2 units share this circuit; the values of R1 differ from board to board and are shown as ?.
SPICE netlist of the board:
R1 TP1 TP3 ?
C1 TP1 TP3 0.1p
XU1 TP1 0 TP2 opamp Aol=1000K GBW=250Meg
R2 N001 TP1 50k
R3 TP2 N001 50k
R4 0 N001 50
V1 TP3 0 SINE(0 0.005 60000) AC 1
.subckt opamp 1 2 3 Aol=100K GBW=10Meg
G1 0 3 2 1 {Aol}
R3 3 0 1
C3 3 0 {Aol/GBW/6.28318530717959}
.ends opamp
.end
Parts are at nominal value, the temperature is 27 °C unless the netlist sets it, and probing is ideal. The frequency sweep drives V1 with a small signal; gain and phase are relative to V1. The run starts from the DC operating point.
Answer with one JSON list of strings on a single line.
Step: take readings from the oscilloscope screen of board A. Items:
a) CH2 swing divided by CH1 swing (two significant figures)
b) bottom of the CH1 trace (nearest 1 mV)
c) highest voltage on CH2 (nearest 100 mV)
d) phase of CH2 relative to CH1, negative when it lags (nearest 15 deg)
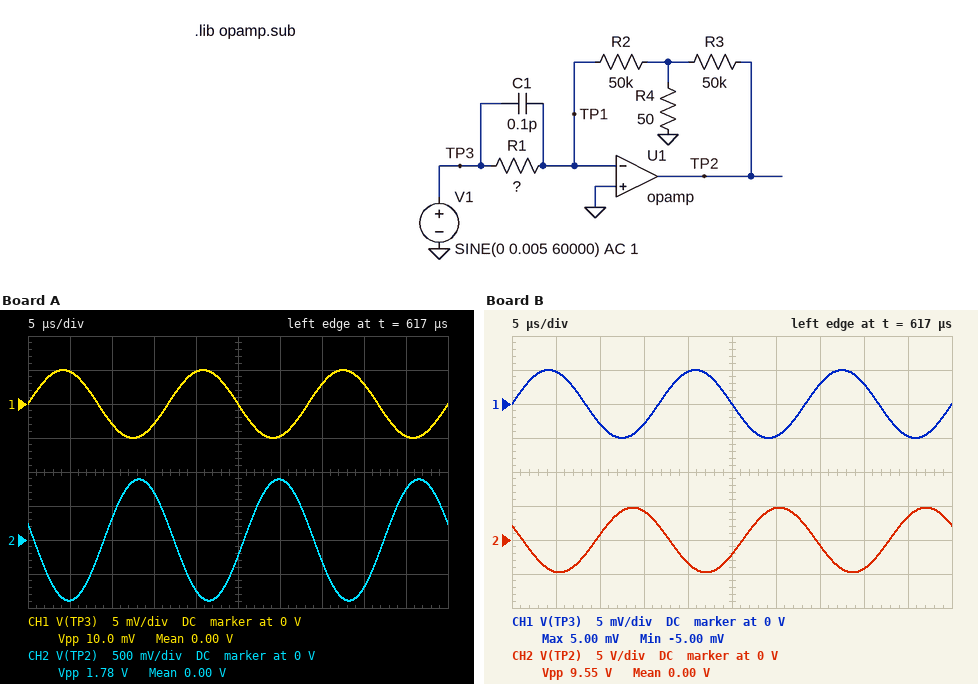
["180", "-5 mV", "900 mV", "165 deg"]
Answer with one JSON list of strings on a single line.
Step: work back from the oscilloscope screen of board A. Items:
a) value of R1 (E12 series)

["270 kΩ"]
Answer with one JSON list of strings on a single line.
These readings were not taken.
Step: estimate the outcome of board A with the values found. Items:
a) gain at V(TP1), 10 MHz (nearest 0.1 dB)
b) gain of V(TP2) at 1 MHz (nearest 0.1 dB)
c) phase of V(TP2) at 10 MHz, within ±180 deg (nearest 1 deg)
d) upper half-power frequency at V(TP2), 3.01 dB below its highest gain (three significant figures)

["-10.5 dB", "31.8 dB", "136 deg", "212 kHz"]
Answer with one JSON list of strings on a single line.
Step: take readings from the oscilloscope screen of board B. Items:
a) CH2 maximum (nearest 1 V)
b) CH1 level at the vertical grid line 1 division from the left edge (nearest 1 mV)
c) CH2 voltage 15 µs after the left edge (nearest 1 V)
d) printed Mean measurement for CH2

["5 V", "5 mV", "4 V", "0.00 V"]
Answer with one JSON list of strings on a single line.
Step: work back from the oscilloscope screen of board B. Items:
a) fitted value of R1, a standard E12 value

["47 kΩ"]
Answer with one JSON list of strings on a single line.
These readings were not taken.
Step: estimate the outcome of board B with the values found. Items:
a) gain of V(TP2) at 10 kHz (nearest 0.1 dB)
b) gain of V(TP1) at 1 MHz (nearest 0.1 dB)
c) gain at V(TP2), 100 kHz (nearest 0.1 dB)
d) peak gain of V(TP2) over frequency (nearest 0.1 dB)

["60.5 dB", "-5.8 dB", "58.3 dB", "60.5 dB"]
